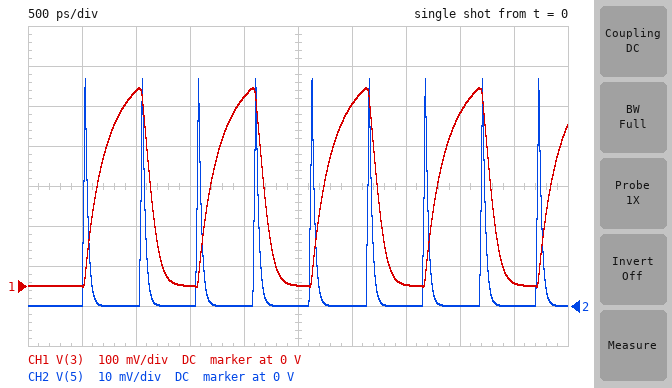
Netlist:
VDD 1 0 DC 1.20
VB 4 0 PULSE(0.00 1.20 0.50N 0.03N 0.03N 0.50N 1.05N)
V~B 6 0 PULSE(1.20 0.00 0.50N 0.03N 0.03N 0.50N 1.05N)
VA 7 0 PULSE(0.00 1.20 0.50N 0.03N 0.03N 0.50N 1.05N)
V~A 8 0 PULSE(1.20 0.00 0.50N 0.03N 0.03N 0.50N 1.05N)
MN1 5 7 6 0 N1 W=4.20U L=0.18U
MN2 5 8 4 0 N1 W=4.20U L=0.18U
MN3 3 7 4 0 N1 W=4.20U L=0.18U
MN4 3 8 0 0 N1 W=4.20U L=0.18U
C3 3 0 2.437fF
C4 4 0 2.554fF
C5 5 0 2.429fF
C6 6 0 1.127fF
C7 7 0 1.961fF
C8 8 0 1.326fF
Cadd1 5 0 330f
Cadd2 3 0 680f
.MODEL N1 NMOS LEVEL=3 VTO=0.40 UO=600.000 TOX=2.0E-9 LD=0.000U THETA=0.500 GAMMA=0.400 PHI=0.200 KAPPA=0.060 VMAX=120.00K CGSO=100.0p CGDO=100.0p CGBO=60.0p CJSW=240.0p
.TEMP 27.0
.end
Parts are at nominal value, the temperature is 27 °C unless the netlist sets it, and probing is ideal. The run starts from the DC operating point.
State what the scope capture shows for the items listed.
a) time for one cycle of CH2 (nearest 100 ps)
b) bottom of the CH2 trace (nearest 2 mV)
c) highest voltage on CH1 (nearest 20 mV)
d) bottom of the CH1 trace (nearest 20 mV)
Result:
500 ps
0 V
500 mV
0 V
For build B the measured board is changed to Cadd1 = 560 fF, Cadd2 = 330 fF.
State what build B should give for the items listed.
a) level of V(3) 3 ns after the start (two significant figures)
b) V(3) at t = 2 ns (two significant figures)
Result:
540 mV
550 mV
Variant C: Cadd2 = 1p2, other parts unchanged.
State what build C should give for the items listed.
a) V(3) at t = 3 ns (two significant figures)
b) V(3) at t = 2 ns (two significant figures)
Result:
360 mV
380 mV
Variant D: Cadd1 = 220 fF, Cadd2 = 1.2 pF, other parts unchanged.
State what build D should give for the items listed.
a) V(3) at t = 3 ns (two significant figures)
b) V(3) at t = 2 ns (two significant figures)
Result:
360 mV
380 mV
